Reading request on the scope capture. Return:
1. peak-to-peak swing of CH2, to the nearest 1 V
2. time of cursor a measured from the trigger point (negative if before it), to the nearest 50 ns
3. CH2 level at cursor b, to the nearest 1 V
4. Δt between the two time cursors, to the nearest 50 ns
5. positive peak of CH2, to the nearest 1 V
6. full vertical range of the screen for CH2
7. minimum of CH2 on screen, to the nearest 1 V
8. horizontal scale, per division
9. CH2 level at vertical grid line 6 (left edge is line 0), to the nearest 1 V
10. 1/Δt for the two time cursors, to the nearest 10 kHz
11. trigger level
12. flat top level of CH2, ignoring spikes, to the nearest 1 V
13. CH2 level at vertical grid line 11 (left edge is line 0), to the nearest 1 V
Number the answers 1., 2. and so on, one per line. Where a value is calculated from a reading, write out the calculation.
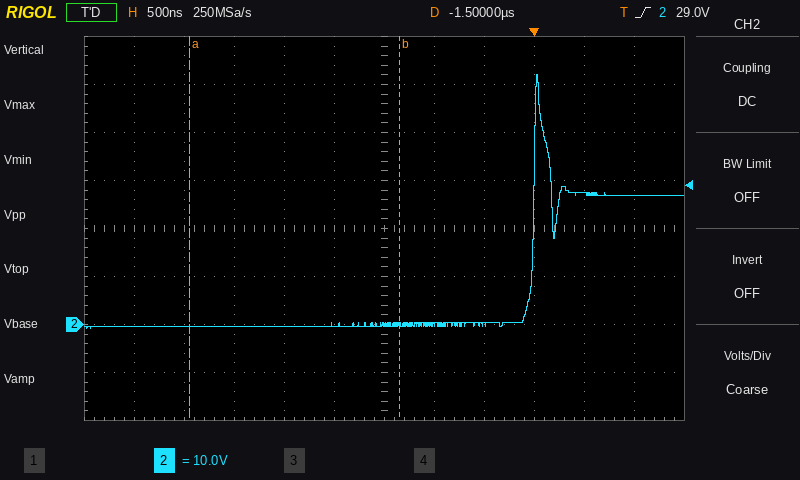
1. 52 V − (-1 V) = 53 V
2. -3.45 µs
3. 0 V
4. 2.10 µs
5. 52 V
6. 80 V
7. -1 V
8. 500 ns
9. 0 V
10. 1 / 2.10 µs ≈ 480 kHz
11. 29.0 V
12. 27 V
13. 27 V
